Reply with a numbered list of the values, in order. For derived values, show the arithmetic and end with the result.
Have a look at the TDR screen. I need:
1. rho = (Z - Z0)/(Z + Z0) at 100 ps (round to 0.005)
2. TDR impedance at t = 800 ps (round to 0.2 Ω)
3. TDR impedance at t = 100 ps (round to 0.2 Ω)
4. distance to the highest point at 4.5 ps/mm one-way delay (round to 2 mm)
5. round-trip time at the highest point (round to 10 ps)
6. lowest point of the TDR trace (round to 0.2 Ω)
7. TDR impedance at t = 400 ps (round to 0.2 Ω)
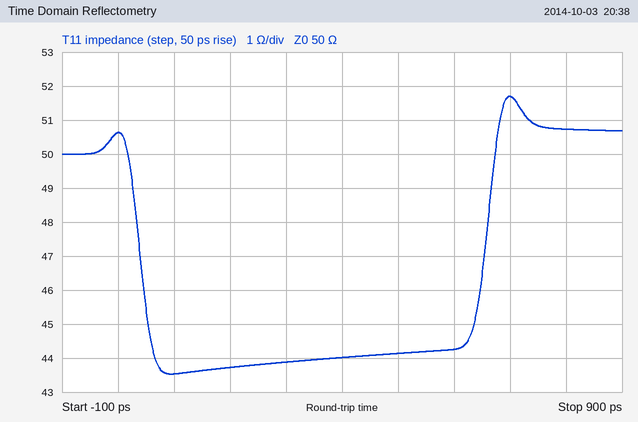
1. (43.6 − 50)/(43.6 + 50) ≈ -0.0684, so -0.070 to the nearest 0.005
2. 50.8 Ω
3. 43.6 Ω
4. 700 ps / 2 / 4.5 ps/mm ≈ 78 mm
5. 700 ps
6. 43.6 Ω
7. 44.0 Ω
